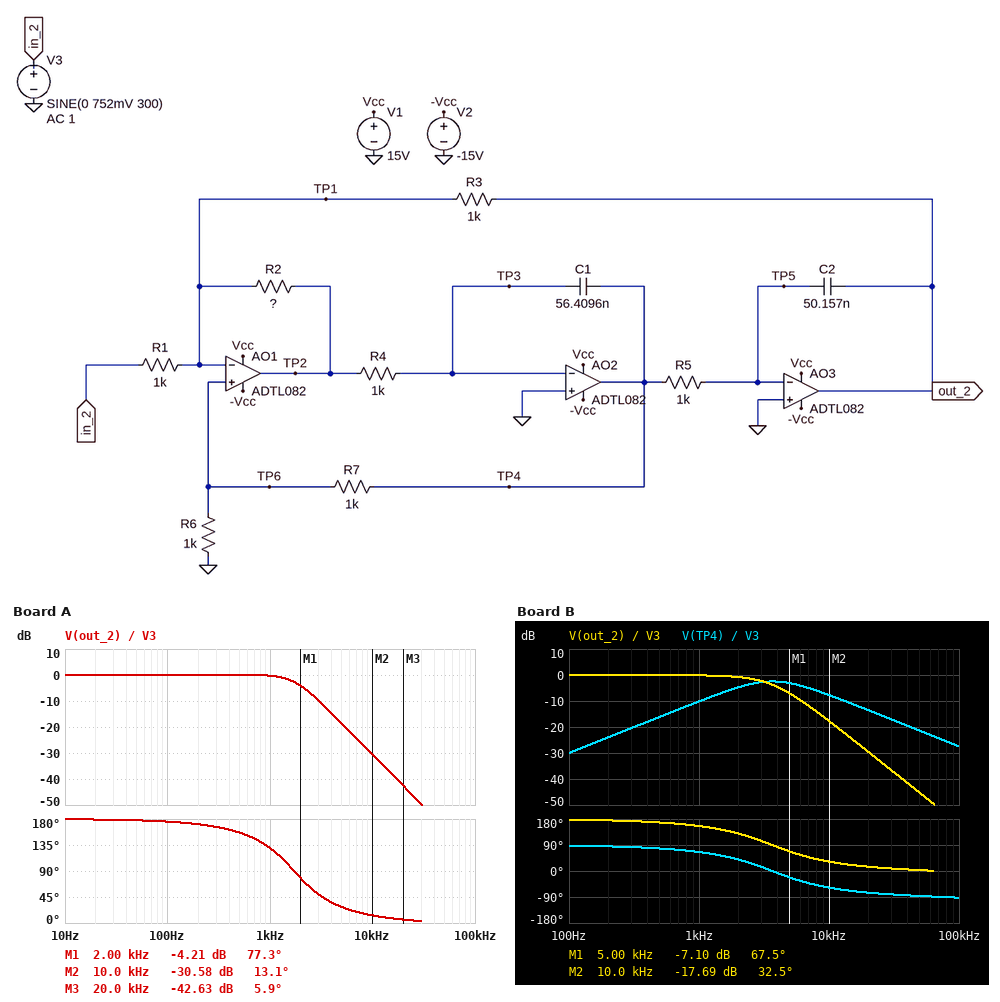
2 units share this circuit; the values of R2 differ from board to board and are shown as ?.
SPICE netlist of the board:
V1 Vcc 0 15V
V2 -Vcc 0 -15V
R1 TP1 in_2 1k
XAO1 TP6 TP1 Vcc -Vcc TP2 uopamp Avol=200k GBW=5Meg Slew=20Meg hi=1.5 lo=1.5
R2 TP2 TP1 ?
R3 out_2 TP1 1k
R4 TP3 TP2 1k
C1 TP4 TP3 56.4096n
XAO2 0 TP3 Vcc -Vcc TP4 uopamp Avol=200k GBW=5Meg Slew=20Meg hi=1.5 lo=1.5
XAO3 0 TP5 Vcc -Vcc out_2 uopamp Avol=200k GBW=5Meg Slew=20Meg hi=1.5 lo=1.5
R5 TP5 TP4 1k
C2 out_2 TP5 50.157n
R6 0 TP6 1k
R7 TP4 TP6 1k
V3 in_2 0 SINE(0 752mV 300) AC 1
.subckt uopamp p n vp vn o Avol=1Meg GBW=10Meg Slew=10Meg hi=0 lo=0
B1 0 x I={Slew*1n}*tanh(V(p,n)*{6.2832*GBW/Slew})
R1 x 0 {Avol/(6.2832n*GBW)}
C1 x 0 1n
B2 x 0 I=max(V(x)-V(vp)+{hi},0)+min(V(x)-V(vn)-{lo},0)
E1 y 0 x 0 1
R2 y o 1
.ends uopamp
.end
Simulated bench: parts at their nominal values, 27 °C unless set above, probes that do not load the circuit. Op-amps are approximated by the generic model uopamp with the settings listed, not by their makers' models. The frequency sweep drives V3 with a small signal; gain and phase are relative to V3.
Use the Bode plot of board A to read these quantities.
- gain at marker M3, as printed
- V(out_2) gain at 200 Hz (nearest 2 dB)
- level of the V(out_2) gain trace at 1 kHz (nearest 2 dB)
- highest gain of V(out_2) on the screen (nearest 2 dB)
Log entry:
-42.63 dB
0 dB
0 dB
0 dB
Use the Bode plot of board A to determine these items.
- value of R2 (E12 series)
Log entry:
330 Ω
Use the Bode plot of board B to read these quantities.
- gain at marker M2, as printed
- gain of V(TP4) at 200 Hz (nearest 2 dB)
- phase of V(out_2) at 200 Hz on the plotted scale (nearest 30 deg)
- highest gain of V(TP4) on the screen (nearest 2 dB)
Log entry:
-17.69 dB
-24 dB
180 deg
-2 dB
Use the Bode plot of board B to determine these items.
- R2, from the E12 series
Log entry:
1.5 kΩ
